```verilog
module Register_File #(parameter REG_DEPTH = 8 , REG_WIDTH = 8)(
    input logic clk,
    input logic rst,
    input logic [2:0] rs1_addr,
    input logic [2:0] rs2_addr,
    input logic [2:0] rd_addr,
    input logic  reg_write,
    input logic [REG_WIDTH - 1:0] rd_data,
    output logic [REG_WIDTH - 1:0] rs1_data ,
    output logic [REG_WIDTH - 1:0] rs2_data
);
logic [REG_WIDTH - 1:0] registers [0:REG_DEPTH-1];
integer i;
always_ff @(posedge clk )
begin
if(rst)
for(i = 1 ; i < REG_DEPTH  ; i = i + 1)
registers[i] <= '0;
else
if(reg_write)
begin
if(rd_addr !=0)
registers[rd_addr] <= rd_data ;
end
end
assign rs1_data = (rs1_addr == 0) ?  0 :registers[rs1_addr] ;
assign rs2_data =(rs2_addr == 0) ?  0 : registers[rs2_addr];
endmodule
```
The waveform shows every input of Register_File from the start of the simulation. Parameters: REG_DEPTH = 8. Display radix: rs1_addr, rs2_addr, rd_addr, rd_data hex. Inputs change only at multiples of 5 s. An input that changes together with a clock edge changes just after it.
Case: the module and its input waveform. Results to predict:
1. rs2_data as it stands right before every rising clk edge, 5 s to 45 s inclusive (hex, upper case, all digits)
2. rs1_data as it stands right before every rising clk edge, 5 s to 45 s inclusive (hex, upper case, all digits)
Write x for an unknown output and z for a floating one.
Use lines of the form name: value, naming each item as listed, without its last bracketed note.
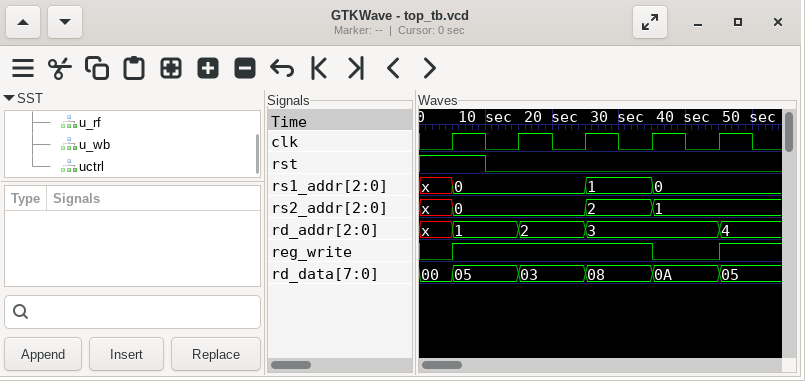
rs2_data as it stands right before every rising clk edge, 5 s to 45 s inclusive: x, 00, 00, 03, 05
rs1_data as it stands right before every rising clk edge, 5 s to 45 s inclusive: x, 00, 00, 05, 00
